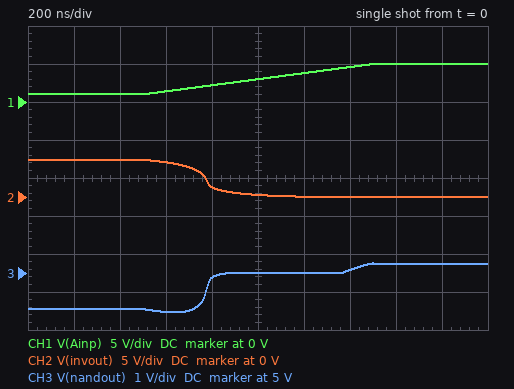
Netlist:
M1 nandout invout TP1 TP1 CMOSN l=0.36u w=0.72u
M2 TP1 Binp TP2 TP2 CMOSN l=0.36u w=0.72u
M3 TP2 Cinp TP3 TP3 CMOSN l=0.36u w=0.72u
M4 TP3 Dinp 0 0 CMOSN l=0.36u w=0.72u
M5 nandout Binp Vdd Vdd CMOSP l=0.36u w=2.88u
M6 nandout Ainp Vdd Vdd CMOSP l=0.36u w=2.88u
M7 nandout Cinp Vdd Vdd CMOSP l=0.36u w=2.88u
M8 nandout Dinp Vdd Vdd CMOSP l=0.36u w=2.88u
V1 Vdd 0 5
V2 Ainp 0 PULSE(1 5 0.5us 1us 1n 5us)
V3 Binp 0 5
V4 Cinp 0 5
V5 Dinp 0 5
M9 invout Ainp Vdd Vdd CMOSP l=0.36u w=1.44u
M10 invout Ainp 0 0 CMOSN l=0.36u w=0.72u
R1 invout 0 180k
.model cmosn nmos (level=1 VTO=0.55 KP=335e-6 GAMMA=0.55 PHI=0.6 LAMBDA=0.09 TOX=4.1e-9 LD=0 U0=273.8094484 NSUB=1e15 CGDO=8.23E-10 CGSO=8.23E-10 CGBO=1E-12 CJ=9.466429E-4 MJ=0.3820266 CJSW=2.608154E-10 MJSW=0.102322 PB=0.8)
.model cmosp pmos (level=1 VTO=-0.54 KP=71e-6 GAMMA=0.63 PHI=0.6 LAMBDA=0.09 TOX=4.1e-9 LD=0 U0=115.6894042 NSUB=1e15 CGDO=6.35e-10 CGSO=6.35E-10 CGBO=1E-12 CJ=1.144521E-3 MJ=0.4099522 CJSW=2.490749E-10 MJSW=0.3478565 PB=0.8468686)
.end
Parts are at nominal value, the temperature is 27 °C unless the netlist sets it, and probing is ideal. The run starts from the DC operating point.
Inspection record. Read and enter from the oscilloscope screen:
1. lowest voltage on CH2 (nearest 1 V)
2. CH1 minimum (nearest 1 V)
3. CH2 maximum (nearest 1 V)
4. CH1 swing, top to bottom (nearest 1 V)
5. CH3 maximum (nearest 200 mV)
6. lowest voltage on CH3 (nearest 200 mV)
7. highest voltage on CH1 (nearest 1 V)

0 V
1 V
5 V
4 V
5.2 V
4.0 V
5 V
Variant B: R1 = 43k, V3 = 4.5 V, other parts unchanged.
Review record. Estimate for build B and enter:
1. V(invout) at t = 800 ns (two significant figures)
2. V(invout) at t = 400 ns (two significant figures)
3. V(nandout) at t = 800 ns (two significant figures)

1.2 V
4.8 V
4.9 V
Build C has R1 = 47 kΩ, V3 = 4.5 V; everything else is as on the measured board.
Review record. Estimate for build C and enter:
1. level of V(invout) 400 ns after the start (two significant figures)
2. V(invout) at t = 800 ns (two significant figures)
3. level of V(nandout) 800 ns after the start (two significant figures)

4.8 V
1.2 V
4.9 V
